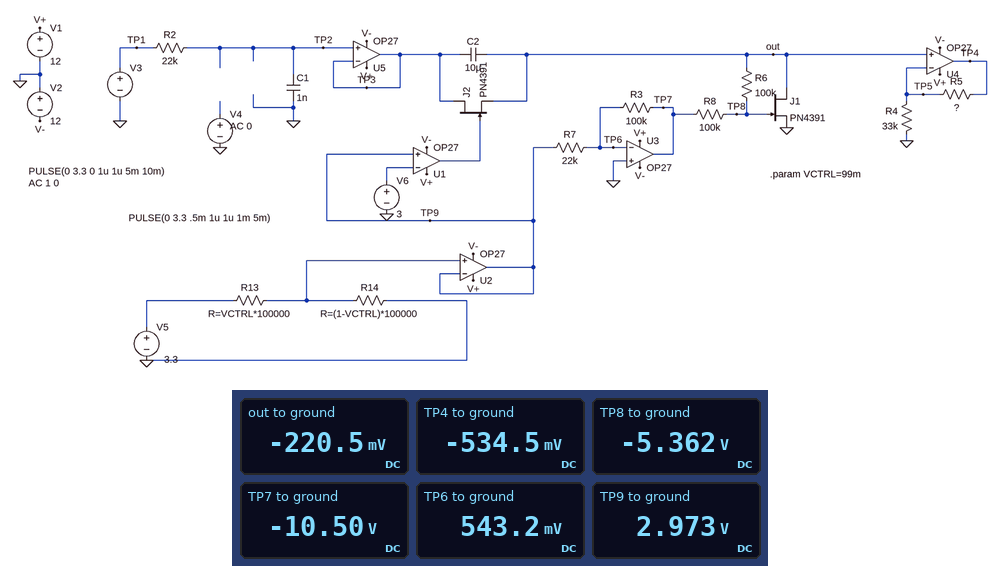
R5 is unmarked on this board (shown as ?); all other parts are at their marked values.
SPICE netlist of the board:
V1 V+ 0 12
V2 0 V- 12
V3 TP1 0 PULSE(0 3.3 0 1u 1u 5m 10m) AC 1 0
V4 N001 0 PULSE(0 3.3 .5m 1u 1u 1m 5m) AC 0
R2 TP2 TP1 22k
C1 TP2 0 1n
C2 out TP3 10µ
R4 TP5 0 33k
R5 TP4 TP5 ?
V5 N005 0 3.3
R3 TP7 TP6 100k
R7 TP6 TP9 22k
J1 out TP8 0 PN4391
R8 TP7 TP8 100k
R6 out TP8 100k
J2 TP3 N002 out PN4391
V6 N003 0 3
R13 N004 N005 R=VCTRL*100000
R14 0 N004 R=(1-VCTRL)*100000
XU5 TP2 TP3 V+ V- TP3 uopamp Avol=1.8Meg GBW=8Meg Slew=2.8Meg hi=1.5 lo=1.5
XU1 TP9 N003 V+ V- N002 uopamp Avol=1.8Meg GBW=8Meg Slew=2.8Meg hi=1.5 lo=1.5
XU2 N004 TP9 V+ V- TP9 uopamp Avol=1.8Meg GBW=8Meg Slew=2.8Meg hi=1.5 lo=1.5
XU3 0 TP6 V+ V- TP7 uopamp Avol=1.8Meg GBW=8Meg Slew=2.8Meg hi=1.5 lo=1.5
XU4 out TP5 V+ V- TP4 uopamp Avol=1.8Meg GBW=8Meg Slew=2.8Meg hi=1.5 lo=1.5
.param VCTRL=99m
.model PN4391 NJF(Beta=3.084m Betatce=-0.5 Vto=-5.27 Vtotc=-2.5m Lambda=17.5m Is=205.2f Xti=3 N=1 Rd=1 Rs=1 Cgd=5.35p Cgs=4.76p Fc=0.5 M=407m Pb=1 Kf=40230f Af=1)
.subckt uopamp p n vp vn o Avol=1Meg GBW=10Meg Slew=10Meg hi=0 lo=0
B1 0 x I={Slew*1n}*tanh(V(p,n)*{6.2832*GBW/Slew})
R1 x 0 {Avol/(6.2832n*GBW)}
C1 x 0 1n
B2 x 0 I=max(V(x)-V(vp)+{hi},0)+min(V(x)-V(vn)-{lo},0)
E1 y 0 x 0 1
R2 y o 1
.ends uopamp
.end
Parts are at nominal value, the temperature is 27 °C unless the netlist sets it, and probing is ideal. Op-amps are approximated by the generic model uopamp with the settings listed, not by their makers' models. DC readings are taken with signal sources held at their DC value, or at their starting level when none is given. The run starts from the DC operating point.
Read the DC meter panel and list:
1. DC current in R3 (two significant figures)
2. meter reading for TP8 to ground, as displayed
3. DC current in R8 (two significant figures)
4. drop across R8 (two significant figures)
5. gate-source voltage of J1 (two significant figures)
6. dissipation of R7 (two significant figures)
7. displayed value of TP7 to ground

110 µA
-5.362 V
51 µA
5.1 V
-5.4 V
270 µW
-10.50 V
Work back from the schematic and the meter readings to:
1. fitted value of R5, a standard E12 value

47 kΩ
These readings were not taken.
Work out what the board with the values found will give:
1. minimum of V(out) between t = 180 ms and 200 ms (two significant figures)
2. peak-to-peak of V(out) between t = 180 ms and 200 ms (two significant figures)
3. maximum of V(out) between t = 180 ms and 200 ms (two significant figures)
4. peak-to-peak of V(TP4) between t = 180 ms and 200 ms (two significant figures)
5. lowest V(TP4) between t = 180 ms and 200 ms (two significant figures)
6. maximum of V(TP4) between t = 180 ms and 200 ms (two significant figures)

-2.1 V
4.2 V
2.1 V
10 V
-5.2 V
5.1 V
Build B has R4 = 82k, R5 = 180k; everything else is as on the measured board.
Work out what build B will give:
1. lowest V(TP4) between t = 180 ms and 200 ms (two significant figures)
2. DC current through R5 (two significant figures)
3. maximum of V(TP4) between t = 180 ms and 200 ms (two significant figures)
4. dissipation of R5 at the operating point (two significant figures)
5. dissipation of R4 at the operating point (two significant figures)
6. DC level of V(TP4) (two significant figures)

-6.8 V
2.7 µA
6.7 V
1.3 µW
590 nW
-700 mV
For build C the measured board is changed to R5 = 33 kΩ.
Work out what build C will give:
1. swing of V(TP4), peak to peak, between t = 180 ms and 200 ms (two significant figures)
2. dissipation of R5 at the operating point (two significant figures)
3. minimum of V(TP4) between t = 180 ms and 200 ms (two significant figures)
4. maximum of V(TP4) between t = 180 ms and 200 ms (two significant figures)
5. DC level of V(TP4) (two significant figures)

8.5 V
1.5 µW
-4.3 V
4.2 V
-440 mV
